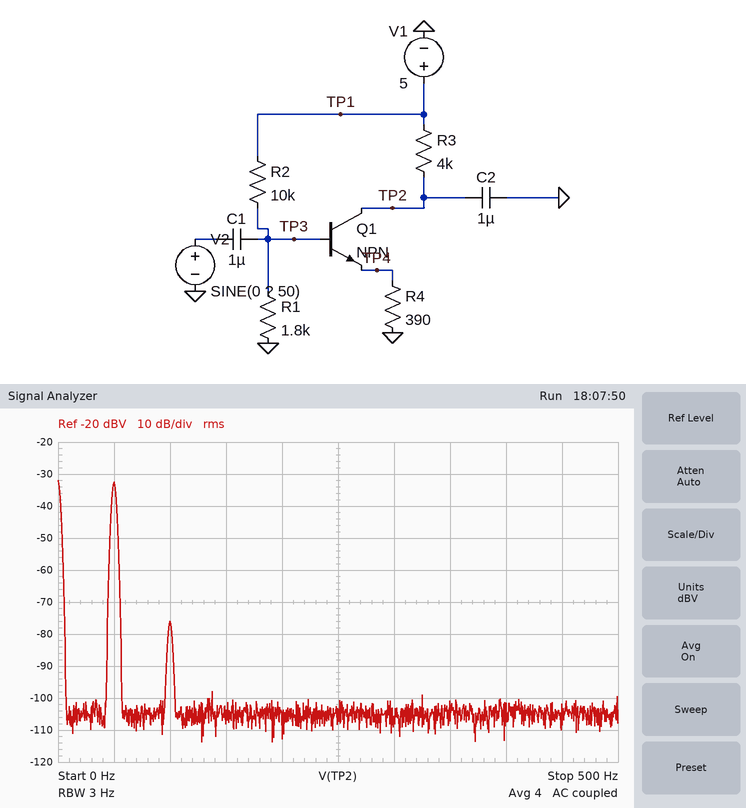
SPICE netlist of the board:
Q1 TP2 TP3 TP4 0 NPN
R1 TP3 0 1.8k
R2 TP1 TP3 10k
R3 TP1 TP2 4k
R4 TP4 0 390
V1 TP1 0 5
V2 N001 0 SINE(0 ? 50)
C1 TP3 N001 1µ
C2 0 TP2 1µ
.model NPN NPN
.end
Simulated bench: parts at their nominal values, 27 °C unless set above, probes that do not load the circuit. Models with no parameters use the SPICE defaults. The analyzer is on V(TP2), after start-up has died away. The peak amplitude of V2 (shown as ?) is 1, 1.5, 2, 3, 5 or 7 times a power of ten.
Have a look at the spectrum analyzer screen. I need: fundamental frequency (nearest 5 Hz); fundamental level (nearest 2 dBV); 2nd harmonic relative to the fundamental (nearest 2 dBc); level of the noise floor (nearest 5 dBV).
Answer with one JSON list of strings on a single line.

["50 Hz", "-32 dBV", "-44 dBc", "-105 dBV"]
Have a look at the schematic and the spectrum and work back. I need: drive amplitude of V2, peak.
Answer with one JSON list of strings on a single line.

["20 mV"]
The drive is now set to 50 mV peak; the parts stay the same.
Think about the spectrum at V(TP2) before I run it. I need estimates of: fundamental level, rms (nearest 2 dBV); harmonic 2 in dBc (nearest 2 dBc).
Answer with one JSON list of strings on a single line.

["-24 dBV", "-36 dBc"]
